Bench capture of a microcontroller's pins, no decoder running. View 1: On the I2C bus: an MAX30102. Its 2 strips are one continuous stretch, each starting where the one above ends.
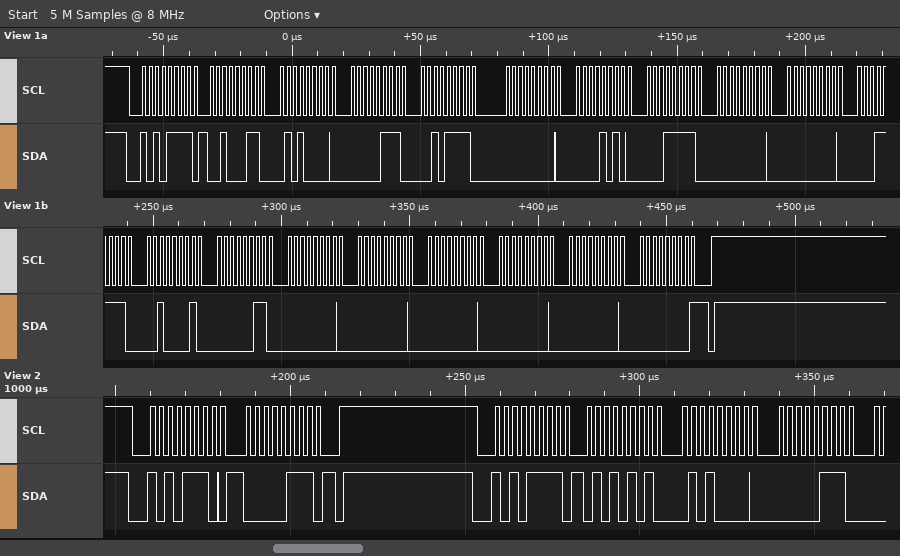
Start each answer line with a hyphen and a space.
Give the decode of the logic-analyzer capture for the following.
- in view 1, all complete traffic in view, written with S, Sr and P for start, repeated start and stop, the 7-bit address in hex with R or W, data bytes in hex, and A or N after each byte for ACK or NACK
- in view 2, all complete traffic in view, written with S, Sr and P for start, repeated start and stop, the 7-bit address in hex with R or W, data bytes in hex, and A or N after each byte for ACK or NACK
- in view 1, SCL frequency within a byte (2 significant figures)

- S 57R A 23 A 50 A 07 A 2F A 00 A 0A A 1F A 00 A 00 A 1F A 21 A 03 A 00 A 00 A 00 A 00 A 00 A 00 N P
- S 57W A 07 A P S 57R A 55 A 50 A 07 A
- 400 kHz
